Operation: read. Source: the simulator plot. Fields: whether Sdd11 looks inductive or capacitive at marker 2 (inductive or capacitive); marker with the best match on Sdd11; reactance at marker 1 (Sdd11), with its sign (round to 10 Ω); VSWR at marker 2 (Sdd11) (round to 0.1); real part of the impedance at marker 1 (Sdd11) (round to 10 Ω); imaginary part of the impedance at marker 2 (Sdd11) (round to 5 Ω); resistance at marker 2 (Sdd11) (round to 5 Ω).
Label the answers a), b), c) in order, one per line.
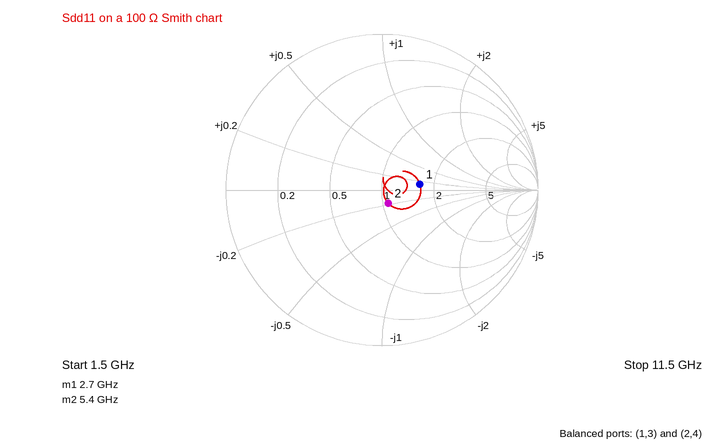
a) capacitive
b) marker 2
c) +10 Ω
d) 1.2
e) 160 Ω
f) -20 Ω
g) 105 Ω
